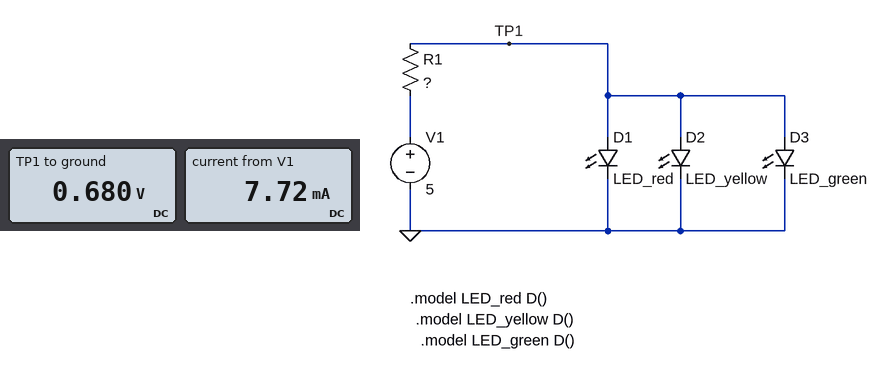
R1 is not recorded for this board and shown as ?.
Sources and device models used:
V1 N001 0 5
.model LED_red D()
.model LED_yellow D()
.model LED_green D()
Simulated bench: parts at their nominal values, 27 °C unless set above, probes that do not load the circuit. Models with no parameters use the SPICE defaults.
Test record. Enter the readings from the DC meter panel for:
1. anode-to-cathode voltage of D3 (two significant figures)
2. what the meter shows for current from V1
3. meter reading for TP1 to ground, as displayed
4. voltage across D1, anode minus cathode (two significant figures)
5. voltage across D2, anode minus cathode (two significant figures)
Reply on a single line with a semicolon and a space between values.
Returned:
680 mV; 7.72 mA; 0.680 V; 680 mV; 680 mV
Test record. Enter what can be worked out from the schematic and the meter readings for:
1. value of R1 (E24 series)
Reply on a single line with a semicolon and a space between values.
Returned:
560 Ω
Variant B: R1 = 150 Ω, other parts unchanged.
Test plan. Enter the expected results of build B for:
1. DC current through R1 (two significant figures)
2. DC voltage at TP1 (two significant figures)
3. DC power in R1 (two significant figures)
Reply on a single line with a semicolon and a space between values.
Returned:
29 mA; 710 mV; 120 mW
